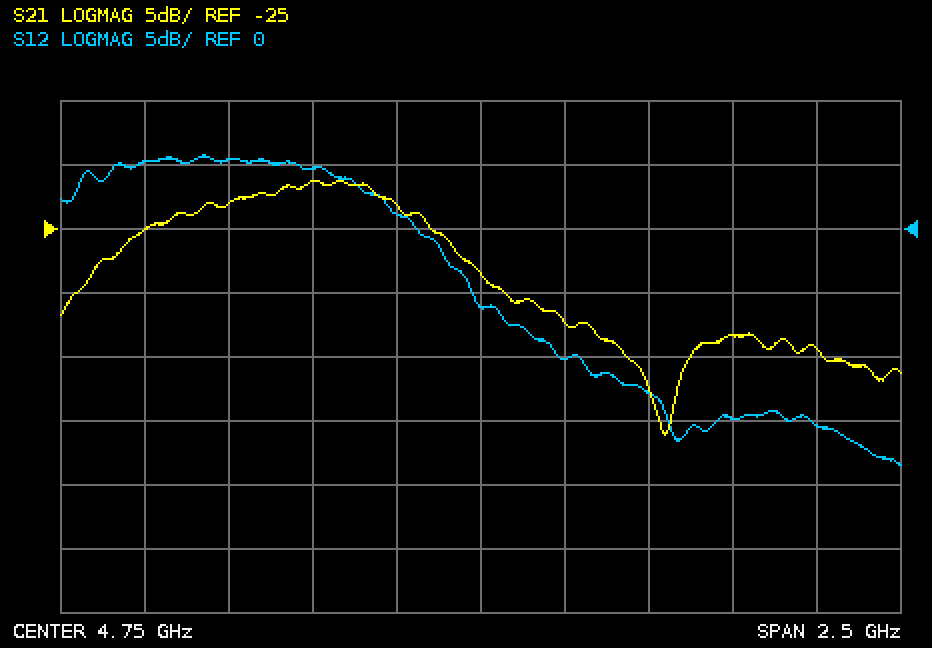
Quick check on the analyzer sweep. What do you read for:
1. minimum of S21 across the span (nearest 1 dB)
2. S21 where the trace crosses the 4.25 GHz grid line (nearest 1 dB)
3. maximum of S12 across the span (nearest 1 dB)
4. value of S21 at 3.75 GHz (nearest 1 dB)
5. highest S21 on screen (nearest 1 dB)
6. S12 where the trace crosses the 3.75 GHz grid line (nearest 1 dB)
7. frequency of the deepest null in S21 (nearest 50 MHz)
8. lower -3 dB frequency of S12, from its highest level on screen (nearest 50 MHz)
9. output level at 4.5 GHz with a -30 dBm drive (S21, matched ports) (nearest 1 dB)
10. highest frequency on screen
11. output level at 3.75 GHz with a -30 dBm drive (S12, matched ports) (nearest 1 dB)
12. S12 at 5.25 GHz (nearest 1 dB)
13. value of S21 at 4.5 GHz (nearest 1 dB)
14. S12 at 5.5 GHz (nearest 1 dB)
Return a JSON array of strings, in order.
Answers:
["-41 dB", "-21 dB", "6 dB", "-25 dB", "-21 dB", "5 dB", "5.30 GHz", "3.55 GHz", "-53 dBm", "6 GHz", "-25 dBm", "-13 dB", "-23 dB", "-15 dB"]
